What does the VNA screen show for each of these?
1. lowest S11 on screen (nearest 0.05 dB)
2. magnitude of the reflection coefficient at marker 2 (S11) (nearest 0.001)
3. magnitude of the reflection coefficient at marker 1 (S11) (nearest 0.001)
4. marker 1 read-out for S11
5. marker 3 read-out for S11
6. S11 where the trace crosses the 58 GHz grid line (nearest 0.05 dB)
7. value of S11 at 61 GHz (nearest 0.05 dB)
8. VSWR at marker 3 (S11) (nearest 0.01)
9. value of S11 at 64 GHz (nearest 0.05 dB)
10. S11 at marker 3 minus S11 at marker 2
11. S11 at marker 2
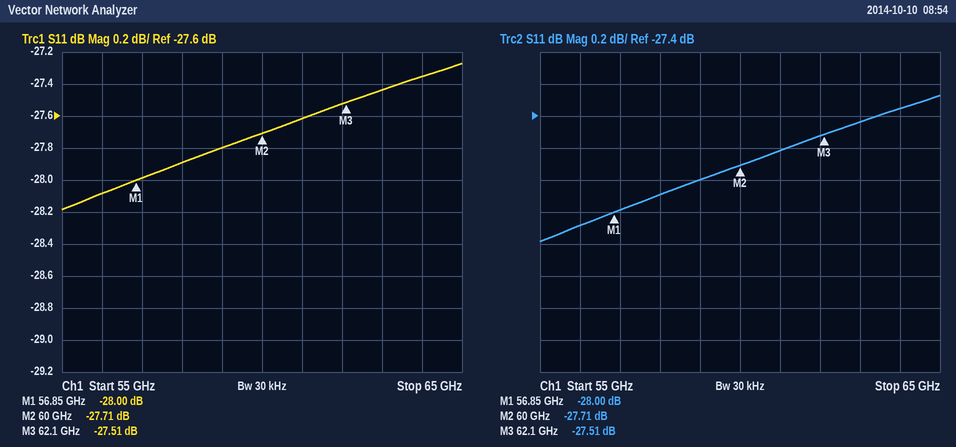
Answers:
-28.20 dB
0.041
0.040
-28.00 dB
-27.51 dB
-27.90 dB
-27.60 dB
1.09
-27.35 dB
0.20 dB
-27.71 dB
